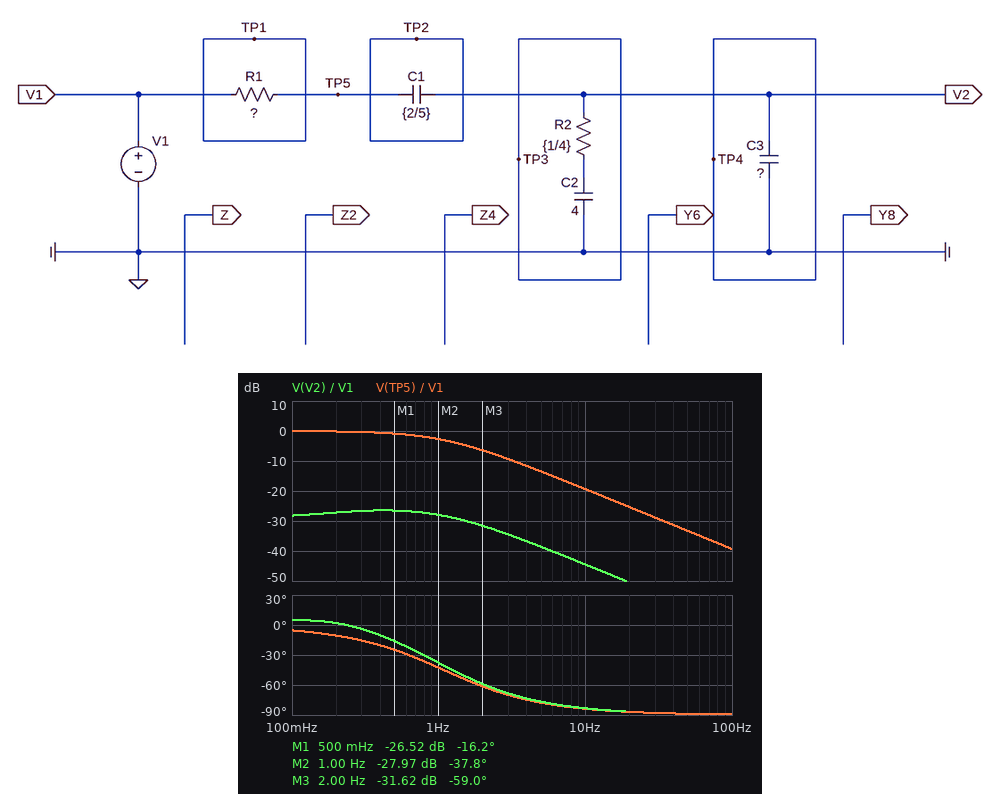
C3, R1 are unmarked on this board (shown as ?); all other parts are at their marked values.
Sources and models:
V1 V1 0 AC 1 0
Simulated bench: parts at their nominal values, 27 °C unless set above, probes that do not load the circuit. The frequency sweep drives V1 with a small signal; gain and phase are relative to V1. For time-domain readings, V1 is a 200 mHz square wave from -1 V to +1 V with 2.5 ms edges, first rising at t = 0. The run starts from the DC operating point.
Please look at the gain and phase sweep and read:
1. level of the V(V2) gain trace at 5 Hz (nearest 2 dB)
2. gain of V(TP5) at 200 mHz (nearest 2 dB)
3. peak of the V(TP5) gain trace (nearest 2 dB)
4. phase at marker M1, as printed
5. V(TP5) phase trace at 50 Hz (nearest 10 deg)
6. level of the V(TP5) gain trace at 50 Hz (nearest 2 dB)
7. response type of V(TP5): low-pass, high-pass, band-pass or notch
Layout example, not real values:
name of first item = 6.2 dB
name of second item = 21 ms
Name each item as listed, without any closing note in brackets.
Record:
level of the V(V2) gain trace at 5 Hz = -38 dB
gain of V(TP5) at 200 mHz = 0 dB
peak of the V(TP5) gain trace = 0 dB
phase at marker M1, as printed = -16.2 deg
V(TP5) phase trace at 50 Hz = -90 deg
level of the V(TP5) gain trace at 50 Hz = -34 dB
response type of V(TP5): low-pass, high-pass, band-pass or notch = low-pass
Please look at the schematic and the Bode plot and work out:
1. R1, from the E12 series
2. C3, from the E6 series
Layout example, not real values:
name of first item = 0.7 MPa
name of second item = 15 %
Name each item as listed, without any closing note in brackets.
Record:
R1, from the E12 series = 0.39 Ω
C3, from the E6 series = 6.8 F
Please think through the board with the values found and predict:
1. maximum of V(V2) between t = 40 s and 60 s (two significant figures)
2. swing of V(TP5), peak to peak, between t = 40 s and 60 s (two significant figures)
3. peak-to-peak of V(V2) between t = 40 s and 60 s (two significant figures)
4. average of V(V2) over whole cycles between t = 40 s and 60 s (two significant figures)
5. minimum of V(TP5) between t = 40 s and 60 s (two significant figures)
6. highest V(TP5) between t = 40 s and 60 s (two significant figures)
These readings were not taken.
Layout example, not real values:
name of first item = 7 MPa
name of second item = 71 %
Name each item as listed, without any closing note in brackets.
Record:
maximum of V(V2) between t = 40 s and 60 s = 90 mV
swing of V(TP5), peak to peak, between t = 40 s and 60 s = 2.0 V
peak-to-peak of V(V2) between t = 40 s and 60 s = 110 mV
average of V(V2) over whole cycles between t = 40 s and 60 s = 36 mV
minimum of V(TP5) between t = 40 s and 60 s = -1.0 V
highest V(TP5) between t = 40 s and 60 s = 1.0 V
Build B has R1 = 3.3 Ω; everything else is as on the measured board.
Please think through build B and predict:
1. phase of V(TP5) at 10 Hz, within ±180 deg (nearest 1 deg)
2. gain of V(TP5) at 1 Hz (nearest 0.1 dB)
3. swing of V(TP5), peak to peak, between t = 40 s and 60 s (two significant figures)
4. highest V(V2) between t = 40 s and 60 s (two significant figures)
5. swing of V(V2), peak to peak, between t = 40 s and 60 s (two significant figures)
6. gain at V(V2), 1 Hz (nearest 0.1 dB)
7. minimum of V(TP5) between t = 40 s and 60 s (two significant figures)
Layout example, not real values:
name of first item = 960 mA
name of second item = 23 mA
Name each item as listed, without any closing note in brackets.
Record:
phase of V(TP5) at 10 Hz, within ±180 deg = -89 deg
gain of V(TP5) at 1 Hz = -18.0 dB
swing of V(TP5), peak to peak, between t = 40 s and 60 s = 1.5 V
highest V(V2) between t = 40 s and 60 s = 67 mV
swing of V(V2), peak to peak, between t = 40 s and 60 s = 62 mV
gain at V(V2), 1 Hz = -43.2 dB
minimum of V(TP5) between t = 40 s and 60 s = -750 mV
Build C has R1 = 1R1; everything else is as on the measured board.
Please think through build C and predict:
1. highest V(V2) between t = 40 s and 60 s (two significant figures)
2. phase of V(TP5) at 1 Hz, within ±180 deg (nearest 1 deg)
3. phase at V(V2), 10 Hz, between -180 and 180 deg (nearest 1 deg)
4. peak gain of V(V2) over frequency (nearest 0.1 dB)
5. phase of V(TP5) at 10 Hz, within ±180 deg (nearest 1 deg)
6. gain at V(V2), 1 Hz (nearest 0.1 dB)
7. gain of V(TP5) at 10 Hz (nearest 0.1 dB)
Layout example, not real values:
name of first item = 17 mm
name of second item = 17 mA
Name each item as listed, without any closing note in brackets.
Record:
highest V(V2) between t = 40 s and 60 s = 78 mV
phase of V(TP5) at 1 Hz, within ±180 deg = -69 deg
phase at V(V2), 10 Hz, between -180 and 180 deg = -87 deg
peak gain of V(V2) over frequency = -28.1 dB
phase of V(TP5) at 10 Hz, within ±180 deg = -88 deg
gain at V(V2), 1 Hz = -34.2 dB
gain of V(TP5) at 10 Hz = -28.3 dB
